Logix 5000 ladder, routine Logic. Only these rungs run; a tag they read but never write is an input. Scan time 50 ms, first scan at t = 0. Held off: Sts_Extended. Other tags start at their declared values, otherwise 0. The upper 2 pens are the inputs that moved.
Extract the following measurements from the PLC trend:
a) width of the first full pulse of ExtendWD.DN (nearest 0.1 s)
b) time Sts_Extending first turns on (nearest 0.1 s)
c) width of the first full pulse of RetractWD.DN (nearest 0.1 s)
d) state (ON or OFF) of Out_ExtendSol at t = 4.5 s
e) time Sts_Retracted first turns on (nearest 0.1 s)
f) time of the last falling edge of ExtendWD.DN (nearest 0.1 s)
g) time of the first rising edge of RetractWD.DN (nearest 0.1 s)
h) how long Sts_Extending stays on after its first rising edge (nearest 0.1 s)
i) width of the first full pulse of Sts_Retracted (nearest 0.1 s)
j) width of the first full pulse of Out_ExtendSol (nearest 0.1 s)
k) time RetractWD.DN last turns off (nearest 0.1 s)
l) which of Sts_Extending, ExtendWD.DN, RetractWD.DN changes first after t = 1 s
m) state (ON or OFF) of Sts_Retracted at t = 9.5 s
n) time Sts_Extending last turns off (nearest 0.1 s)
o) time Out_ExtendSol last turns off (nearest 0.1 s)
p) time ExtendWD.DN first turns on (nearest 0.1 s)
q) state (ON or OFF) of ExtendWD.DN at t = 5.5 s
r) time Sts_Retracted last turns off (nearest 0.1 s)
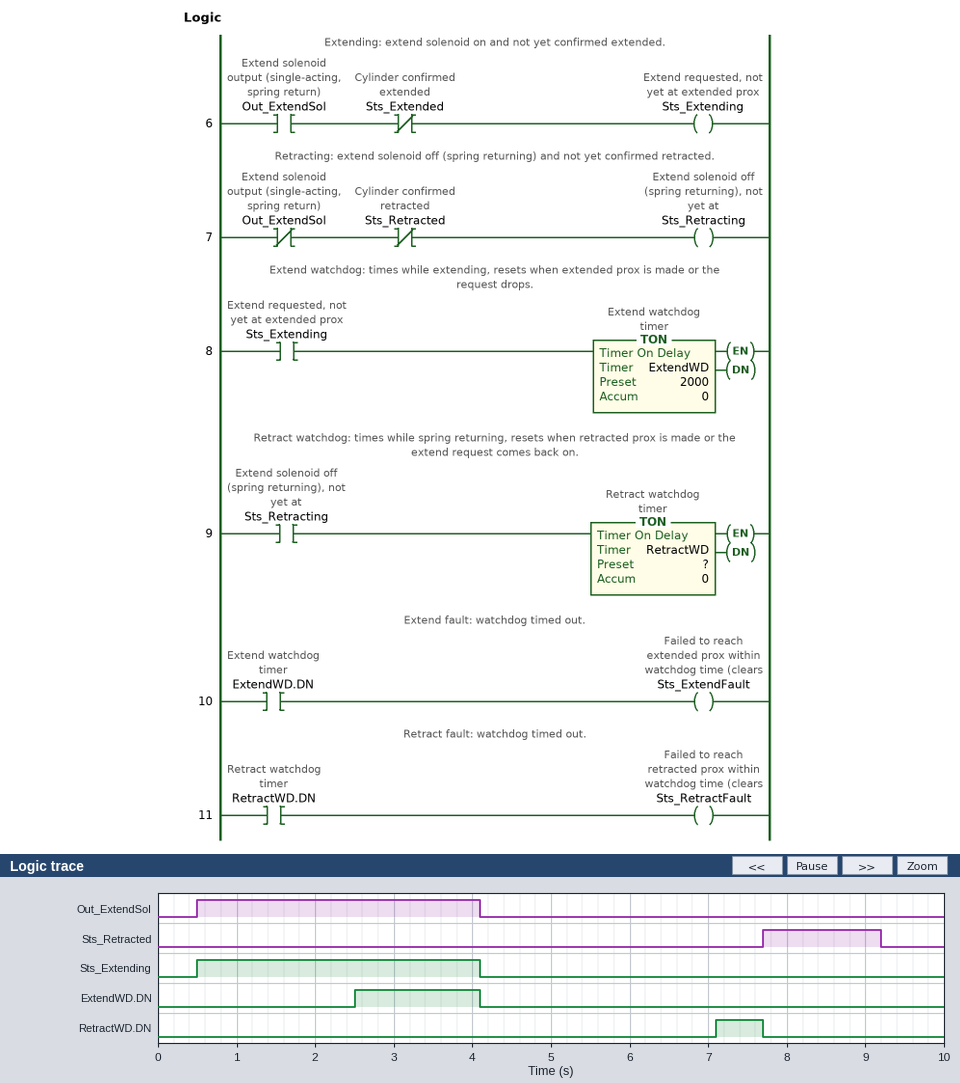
1.6 s
0.5 s
0.6 s
OFF
7.7 s
4.1 s
7.1 s
3.6 s
1.5 s
3.6 s
7.7 s
ExtendWD.DN
OFF
4.1 s
4.1 s
2.5 s
OFF
9.2 s
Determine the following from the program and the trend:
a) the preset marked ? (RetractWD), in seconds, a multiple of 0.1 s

3.0 s
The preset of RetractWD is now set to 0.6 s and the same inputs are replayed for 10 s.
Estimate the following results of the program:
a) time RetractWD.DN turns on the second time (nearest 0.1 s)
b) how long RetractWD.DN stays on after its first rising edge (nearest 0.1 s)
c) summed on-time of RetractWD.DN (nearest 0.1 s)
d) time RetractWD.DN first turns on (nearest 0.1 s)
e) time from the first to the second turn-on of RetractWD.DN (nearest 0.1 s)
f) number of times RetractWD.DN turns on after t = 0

9.8 s
3.0 s
3.2 s
4.7 s
5.1 s
2
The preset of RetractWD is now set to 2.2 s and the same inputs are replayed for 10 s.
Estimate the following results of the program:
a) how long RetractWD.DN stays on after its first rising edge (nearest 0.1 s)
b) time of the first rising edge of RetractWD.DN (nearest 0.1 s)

1.4 s
6.3 s
